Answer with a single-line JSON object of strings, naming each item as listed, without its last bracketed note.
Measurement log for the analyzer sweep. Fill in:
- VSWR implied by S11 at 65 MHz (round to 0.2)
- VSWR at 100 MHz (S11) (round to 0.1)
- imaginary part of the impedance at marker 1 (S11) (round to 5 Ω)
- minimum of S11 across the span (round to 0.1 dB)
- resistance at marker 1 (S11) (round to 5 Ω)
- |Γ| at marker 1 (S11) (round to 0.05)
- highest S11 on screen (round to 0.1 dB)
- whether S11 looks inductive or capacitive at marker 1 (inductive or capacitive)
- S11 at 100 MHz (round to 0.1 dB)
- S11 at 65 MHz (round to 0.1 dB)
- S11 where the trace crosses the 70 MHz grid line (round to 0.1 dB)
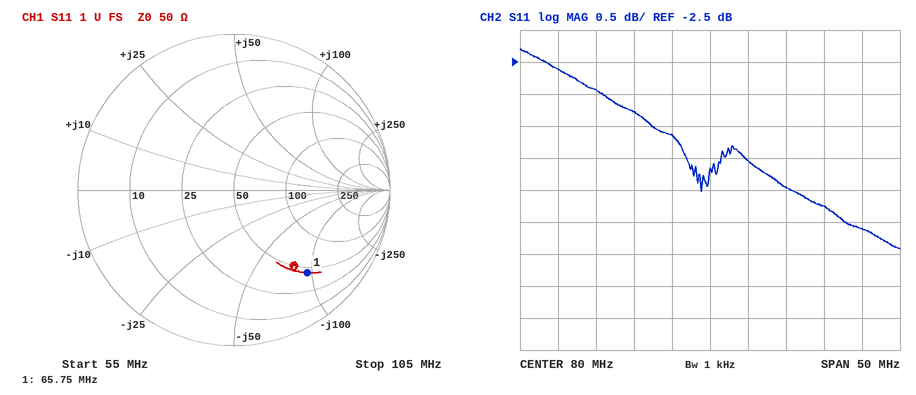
{"VSWR implied by S11 at 65 MHz": "6.0", "VSWR at 100 MHz (S11)": "3.5", "imaginary part of the impedance at marker 1 (S11)": "-95 Ω", "minimum of S11 across the span": "-5.4 dB", "resistance at marker 1 (S11)": "45 Ω", "|Γ| at marker 1 (S11)": "0.70", "highest S11 on screen": "-2.3 dB", "whether S11 looks inductive or capacitive at marker 1": "capacitive", "S11 at 100 MHz": "-5.1 dB", "S11 at 65 MHz": "-2.9 dB", "S11 where the trace crosses the 70 MHz grid line": "-3.3 dB"}
